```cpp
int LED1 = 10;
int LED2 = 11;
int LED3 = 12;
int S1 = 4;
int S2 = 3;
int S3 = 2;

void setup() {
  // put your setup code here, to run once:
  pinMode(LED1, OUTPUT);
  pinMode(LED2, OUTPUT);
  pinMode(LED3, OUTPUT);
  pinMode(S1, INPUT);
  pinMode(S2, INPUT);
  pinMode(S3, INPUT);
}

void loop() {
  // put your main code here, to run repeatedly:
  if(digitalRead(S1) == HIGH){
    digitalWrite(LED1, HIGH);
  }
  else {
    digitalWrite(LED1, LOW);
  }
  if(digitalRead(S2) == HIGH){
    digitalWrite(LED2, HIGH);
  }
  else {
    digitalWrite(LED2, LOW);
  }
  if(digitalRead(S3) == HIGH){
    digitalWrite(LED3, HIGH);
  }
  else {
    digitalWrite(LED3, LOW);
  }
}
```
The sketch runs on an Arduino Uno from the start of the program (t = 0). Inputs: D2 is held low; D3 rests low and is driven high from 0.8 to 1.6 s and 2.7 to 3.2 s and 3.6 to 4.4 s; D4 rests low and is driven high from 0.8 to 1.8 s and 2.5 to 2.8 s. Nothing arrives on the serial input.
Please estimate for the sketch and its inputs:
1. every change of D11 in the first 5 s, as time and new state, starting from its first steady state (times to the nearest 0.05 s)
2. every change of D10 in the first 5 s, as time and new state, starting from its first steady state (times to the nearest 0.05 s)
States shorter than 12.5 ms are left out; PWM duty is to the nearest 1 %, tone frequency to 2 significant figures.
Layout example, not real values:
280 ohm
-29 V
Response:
0 s low; 0.8 s high; 1.6 s low; 2.7 s high; 3.2 s low; 3.6 s high; 4.4 s low
0 s low; 0.8 s high; 1.8 s low; 2.5 s high; 2.8 s low
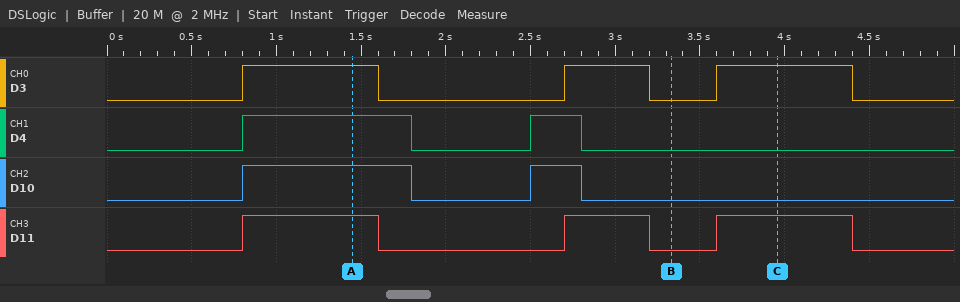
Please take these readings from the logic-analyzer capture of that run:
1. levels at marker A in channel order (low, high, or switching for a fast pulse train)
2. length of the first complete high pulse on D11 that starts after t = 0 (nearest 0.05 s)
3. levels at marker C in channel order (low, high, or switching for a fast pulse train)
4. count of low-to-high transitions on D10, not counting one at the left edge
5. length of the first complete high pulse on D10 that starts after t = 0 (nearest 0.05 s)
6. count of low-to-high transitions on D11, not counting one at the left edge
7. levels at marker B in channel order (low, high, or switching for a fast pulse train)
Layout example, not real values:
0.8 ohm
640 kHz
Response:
D3 high, D4 high, D10 high, D11 high
0.80 s
D3 high, D4 low, D10 low, D11 high
2
1.00 s
3
D3 low, D4 low, D10 low, D11 low
